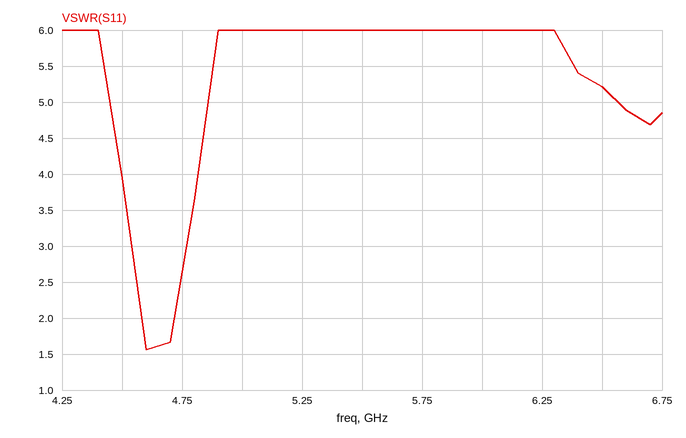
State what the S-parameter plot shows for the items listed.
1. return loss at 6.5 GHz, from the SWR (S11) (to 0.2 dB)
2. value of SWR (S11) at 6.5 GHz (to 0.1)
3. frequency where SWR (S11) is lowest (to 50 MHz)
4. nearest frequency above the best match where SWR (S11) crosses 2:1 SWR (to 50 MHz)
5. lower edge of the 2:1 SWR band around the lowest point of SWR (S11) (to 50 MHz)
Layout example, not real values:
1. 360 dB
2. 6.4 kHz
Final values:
1. 3.4 dB
2. 5.2
3. 4.60 GHz
4. 4.70 GHz
5. 4.60 GHz
